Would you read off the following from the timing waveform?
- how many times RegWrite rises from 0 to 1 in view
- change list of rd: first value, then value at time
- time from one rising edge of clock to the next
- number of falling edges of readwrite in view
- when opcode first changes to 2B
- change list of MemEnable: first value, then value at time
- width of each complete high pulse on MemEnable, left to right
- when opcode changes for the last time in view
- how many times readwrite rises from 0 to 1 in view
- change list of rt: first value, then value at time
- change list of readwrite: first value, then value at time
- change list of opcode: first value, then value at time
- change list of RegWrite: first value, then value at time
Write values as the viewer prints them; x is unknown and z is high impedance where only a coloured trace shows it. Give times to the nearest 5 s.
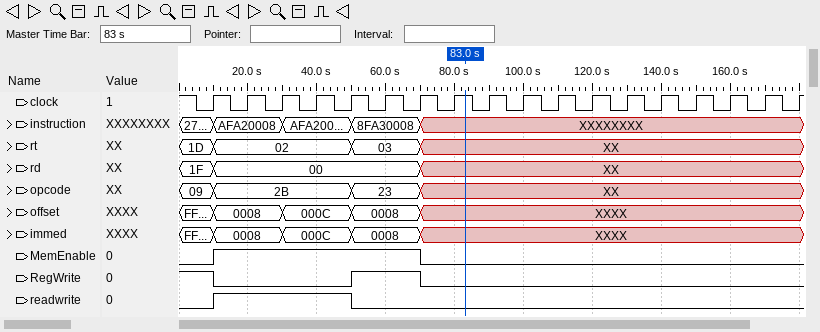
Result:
1
1F, 00 at 10 s, XX at 70 s
10 s
1
10 s
0, 1 at 10 s, 0 at 70 s
60 s
70 s
1
1D, 02 at 10 s, 03 at 50 s, XX at 70 s
0, 1 at 10 s, 0 at 50 s
09, 2B at 10 s, 23 at 50 s, XX at 70 s
1, 0 at 10 s, 1 at 50 s, 0 at 70 s
